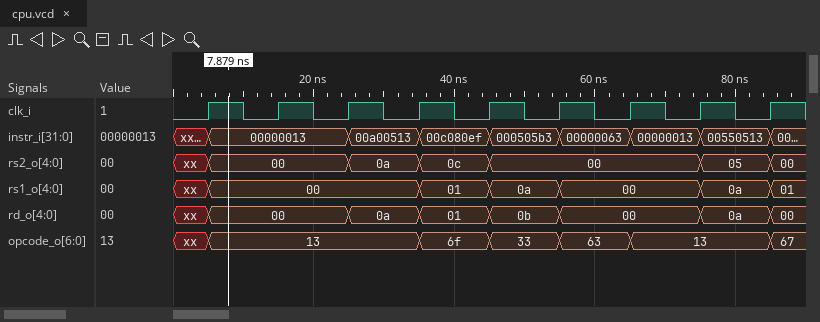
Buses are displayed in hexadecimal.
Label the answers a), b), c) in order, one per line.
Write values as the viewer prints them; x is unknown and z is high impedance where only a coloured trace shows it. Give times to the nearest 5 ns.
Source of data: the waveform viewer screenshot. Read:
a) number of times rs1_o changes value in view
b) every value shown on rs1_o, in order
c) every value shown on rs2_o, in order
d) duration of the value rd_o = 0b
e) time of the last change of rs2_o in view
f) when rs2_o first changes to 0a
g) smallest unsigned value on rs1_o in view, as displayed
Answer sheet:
a) 6
b) xx, 00, 01, 0a, 00, 0a, 01
c) xx, 00, 0a, 0c, 00, 05, 00
d) 10 ns
e) 85 ns
f) 25 ns
g) 00
